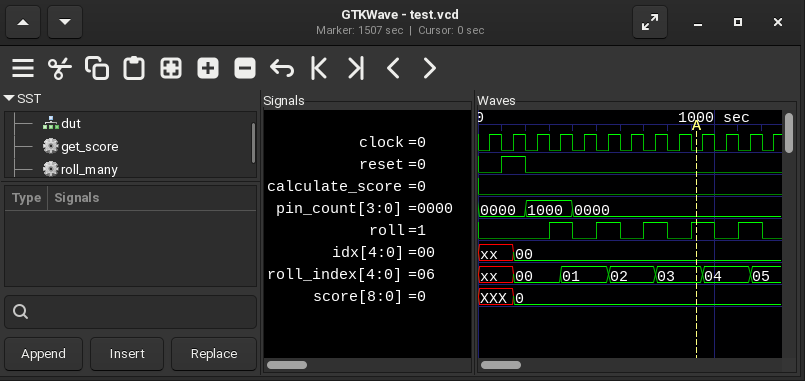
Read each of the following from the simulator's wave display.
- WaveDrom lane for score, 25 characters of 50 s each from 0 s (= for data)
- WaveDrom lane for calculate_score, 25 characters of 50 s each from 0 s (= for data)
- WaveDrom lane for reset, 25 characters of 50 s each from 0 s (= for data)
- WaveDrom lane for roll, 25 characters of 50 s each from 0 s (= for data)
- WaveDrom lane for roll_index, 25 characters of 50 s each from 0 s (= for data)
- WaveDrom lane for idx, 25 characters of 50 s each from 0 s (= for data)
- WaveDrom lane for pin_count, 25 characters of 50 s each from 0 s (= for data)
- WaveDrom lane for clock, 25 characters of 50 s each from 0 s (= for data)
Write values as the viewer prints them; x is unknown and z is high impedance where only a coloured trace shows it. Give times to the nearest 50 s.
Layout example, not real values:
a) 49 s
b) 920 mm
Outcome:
a) {name: 'score', wave: 'x..=.....................', data: '0'}
b) {name: 'calculate_score', wave: '0........................'}
c) {name: 'reset', wave: '0.1.0....................'}
d) {name: 'roll', wave: '0.....1.0.1.0.1.0.1.0.1.0'}
e) {name: 'roll_index', wave: 'x..=...=...=...=...=...=.', data: '00 01 02 03 04 05'}
f) {name: 'idx', wave: 'x..=.....................', data: '00'}
g) {name: 'pin_count', wave: '=...=...=................', data: '0000 1000 0000'}
h) {name: 'clock', wave: '0101010101010101010101010'}
